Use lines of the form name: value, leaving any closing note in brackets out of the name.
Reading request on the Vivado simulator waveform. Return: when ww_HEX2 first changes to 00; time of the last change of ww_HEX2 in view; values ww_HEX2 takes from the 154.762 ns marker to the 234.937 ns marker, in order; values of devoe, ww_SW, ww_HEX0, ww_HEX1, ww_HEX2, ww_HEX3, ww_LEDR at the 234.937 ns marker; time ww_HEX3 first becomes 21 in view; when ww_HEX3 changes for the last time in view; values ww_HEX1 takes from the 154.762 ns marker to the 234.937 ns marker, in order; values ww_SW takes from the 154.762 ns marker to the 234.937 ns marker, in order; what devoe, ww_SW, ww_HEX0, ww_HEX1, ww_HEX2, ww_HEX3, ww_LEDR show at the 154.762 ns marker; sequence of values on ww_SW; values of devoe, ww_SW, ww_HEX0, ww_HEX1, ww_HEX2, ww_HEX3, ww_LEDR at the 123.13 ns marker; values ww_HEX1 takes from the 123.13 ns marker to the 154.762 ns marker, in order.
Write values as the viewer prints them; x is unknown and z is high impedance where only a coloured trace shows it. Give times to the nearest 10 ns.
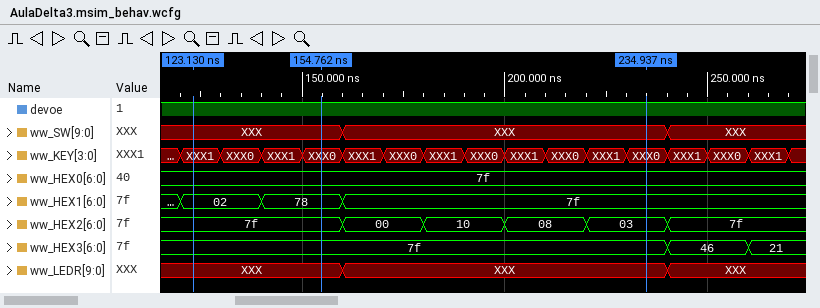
when ww_HEX2 first changes to 00: 160 ns
time of the last change of ww_HEX2 in view: 240 ns
values ww_HEX2 takes from the 154.762 ns marker to the 234.937 ns marker, in order: 7f, 00, 10, 08, 03
values of devoe, ww_SW, ww_HEX0, ww_HEX1, ww_HEX2, ww_HEX3, ww_LEDR at the 234.937 ns marker: devoe=1, ww_SW=XXX, ww_HEX0=7f, ww_HEX1=7f, ww_HEX2=03, ww_HEX3=7f, ww_LEDR=XXX
time ww_HEX3 first becomes 21 in view: 260 ns
when ww_HEX3 changes for the last time in view: 260 ns
values ww_HEX1 takes from the 154.762 ns marker to the 234.937 ns marker, in order: 78, 7f
values ww_SW takes from the 154.762 ns marker to the 234.937 ns marker, in order: XXX, XXX
what devoe, ww_SW, ww_HEX0, ww_HEX1, ww_HEX2, ww_HEX3, ww_LEDR show at the 154.762 ns marker: devoe=1, ww_SW=XXX, ww_HEX0=7f, ww_HEX1=78, ww_HEX2=7f, ww_HEX3=7f, ww_LEDR=XXX
sequence of values on ww_SW: XXX, XXX, XXX
values of devoe, ww_SW, ww_HEX0, ww_HEX1, ww_HEX2, ww_HEX3, ww_LEDR at the 123.13 ns marker: devoe=1, ww_SW=XXX, ww_HEX0=7f, ww_HEX1=02, ww_HEX2=7f, ww_HEX3=7f, ww_LEDR=XXX
values ww_HEX1 takes from the 123.13 ns marker to the 154.762 ns marker, in order: 02, 78
